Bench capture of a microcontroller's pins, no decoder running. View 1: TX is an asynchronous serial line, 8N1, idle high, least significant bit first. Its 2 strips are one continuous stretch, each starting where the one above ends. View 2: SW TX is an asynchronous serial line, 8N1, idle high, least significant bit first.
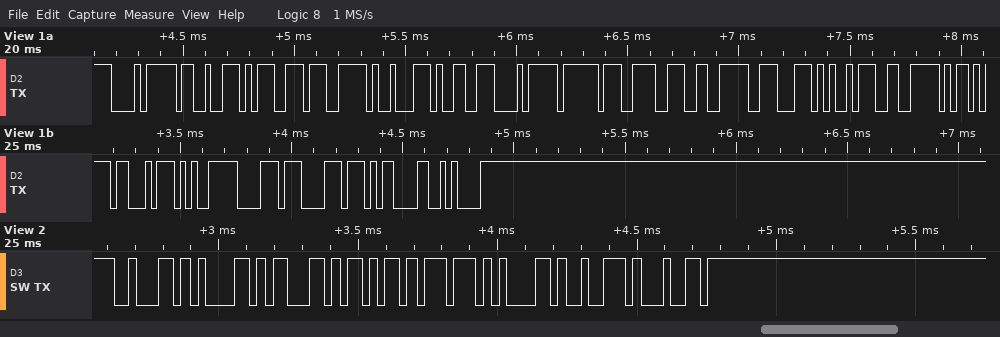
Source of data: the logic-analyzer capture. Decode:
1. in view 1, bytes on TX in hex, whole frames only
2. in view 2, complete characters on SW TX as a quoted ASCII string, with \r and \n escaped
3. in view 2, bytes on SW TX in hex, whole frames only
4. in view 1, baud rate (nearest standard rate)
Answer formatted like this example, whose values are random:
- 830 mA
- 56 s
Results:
- E8 93 9D E7 89 99 E8 BF 9E E6 8E A5 E6 AD A3 E5 B8 B8 0D 0A
- "backward"
- 62 61 63 6B 77 61 72 64
- 38400 baud
